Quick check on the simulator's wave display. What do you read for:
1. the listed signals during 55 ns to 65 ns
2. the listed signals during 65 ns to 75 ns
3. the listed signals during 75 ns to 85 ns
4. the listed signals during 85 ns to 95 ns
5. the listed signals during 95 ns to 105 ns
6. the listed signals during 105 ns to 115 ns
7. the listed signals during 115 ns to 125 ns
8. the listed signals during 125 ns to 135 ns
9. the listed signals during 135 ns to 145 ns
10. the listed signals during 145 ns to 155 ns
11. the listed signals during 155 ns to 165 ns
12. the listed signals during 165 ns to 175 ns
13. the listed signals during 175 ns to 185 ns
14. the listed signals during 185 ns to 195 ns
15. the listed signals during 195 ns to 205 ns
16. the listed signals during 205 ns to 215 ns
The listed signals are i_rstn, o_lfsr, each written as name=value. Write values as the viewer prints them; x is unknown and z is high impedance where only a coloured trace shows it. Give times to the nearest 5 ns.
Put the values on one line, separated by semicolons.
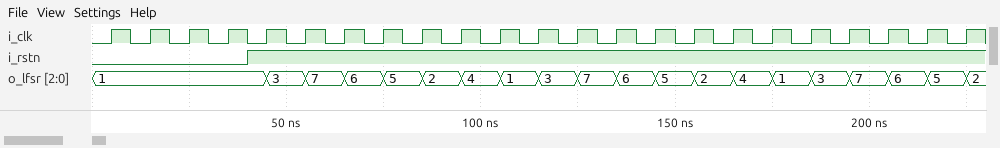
i_rstn=1, o_lfsr=7; i_rstn=1, o_lfsr=6; i_rstn=1, o_lfsr=5; i_rstn=1, o_lfsr=2; i_rstn=1, o_lfsr=4; i_rstn=1, o_lfsr=1; i_rstn=1, o_lfsr=3; i_rstn=1, o_lfsr=7; i_rstn=1, o_lfsr=6; i_rstn=1, o_lfsr=5; i_rstn=1, o_lfsr=2; i_rstn=1, o_lfsr=4; i_rstn=1, o_lfsr=1; i_rstn=1, o_lfsr=3; i_rstn=1, o_lfsr=7; i_rstn=1, o_lfsr=6
